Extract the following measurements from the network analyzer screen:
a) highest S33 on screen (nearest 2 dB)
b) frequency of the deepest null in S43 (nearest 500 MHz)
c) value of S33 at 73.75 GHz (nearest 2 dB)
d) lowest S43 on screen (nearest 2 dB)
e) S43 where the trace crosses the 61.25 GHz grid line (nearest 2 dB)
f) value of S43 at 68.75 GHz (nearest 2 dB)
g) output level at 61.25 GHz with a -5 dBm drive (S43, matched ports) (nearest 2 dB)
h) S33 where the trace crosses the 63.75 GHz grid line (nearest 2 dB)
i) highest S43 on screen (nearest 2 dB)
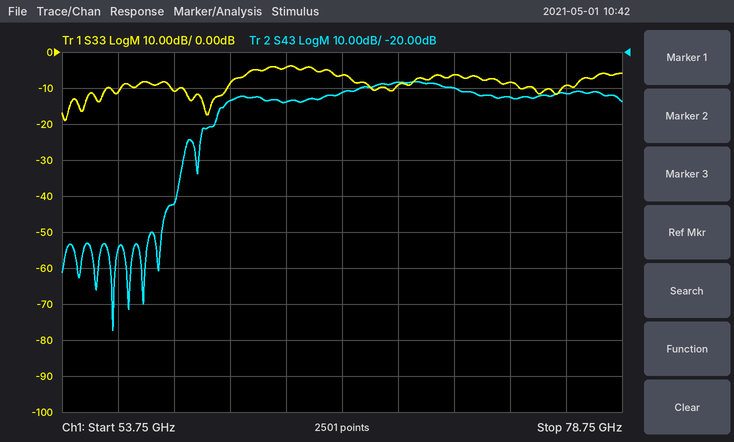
-4 dB
56.0 GHz
-8 dB
-98 dB
-34 dB
-28 dB
-38 dBm
-4 dB
-28 dB
